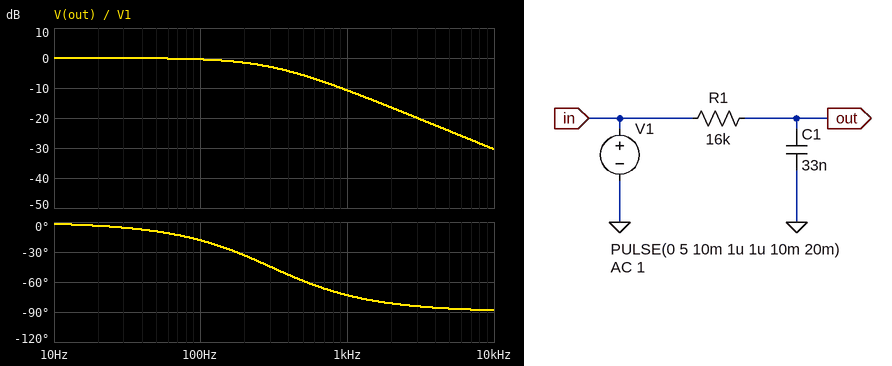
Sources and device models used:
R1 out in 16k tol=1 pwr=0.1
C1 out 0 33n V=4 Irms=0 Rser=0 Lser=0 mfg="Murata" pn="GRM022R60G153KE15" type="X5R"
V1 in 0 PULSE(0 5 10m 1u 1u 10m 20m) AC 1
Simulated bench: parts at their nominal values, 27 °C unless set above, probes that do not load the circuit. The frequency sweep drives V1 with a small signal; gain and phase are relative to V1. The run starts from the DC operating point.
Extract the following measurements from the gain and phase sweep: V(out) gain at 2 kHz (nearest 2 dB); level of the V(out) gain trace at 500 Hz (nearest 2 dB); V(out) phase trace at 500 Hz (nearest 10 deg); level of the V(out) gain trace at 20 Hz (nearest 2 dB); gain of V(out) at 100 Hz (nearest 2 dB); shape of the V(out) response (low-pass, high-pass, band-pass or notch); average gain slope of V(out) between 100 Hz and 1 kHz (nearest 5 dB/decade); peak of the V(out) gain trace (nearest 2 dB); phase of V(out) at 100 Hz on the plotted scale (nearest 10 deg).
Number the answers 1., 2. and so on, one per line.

1. -16 dB
2. -6 dB
3. -60 deg
4. 0 dB
5. 0 dB
6. low-pass
7. -10 dB/decade
8. 0 dB
9. -20 deg
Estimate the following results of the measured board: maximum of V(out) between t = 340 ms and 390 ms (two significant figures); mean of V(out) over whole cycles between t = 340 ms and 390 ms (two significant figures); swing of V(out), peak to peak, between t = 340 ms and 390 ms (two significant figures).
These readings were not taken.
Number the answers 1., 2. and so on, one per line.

1. 5.0 V
2. 2.5 V
3. 5.0 V
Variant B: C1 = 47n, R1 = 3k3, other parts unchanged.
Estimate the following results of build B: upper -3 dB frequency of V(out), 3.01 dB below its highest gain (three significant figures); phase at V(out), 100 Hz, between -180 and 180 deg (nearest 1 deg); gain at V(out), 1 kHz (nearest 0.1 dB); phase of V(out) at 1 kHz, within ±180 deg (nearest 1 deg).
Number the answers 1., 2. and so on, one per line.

1. 1.03 kHz
2. -6 deg
3. -2.9 dB
4. -44 deg
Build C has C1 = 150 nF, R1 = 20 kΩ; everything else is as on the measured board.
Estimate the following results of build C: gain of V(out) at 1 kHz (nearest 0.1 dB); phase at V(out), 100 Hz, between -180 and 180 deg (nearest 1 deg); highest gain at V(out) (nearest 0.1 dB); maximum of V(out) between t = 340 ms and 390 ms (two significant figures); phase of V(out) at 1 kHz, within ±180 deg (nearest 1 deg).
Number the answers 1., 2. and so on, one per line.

1. -25.5 dB
2. -62 deg
3. 0 dB
4. 4.8 V
5. -87 deg
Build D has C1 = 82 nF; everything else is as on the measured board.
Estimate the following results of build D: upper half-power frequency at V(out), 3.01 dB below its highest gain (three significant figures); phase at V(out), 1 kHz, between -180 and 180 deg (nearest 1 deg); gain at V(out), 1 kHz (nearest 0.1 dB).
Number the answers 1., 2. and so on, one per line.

1. 121 Hz
2. -83 deg
3. -18.4 dB
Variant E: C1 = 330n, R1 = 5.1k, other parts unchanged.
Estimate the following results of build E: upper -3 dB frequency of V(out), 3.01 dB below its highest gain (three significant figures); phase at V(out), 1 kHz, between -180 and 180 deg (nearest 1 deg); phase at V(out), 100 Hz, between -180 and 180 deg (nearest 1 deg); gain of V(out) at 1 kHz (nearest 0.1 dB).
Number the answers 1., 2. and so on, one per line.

1. 94.6 Hz
2. -85 deg
3. -47 deg
4. -20.5 dB
